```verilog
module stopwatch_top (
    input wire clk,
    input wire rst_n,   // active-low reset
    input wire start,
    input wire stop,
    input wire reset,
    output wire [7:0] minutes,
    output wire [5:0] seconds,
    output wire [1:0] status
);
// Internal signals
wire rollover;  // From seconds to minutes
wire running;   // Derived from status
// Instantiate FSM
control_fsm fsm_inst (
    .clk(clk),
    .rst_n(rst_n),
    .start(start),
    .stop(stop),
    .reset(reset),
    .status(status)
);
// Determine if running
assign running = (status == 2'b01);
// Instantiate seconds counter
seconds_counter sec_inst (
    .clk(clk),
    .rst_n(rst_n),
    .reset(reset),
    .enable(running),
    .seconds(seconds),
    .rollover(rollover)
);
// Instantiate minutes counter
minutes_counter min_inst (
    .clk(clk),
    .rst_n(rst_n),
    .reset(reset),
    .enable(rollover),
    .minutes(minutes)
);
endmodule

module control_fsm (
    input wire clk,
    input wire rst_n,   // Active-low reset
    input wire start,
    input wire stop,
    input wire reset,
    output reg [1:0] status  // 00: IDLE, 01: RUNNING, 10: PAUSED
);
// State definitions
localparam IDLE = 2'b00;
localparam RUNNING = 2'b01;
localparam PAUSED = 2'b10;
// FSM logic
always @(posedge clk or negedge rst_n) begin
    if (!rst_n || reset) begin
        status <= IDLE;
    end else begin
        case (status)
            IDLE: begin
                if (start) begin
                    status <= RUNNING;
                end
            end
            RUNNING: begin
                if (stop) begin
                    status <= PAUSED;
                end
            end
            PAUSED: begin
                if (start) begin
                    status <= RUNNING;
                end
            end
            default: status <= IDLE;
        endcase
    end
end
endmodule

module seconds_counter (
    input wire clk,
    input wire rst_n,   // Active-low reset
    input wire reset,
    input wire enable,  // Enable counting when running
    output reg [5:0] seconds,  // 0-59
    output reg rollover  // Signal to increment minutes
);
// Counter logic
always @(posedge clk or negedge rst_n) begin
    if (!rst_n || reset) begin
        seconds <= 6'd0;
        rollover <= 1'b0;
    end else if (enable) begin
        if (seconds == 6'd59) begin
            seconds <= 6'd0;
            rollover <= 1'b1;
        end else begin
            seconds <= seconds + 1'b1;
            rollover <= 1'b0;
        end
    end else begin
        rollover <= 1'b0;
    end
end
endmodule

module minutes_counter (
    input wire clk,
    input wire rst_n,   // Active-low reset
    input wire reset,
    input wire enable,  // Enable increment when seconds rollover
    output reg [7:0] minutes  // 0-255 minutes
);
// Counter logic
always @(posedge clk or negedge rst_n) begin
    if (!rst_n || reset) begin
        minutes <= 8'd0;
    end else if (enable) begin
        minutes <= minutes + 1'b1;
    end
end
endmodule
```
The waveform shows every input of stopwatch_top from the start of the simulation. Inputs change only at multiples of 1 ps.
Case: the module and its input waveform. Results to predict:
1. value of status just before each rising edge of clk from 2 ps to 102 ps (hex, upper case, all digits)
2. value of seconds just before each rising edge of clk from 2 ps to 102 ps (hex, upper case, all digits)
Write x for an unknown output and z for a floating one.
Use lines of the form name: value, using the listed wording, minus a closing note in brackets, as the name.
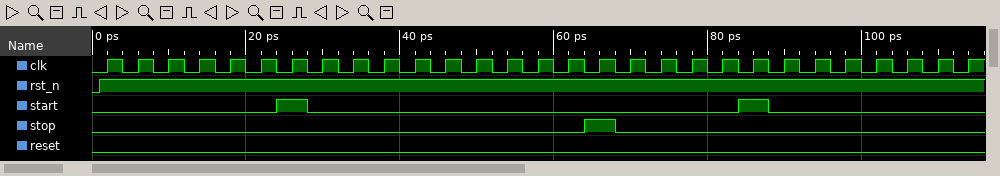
value of status just before each rising edge of clk from 2 ps to 102 ps: 0, 0, 0, 0, 0, 0, 0, 1, 1, 1, 1, 1, 1, 1, 1, 1, 1, 2, 2, 2, 2, 2, 1, 1, 1, 1
value of seconds just before each rising edge of clk from 2 ps to 102 ps: 00, 00, 00, 00, 00, 00, 00, 00, 01, 02, 03, 04, 05, 06, 07, 08, 09, 0A, 0A, 0A, 0A, 0A, 0A, 0B, 0C, 0D
